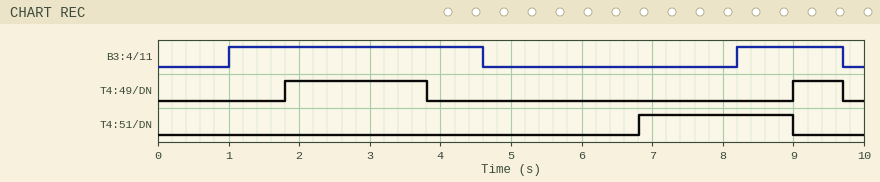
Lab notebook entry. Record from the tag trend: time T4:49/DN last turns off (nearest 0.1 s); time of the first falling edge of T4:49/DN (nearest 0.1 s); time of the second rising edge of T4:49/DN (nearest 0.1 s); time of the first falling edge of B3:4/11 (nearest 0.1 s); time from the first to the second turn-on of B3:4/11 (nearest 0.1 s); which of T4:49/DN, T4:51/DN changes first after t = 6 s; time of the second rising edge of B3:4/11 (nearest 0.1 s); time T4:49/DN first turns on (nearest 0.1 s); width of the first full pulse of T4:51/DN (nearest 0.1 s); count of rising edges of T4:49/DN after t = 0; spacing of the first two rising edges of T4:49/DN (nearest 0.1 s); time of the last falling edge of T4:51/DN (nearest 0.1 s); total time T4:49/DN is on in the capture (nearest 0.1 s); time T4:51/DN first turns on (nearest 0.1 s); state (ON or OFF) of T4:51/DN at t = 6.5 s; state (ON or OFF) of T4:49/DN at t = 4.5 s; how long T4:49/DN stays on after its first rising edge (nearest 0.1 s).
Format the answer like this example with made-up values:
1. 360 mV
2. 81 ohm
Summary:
1. 9.7 s
2. 3.8 s
3. 9.0 s
4. 4.6 s
5. 7.2 s
6. T4:51/DN
7. 8.2 s
8. 1.8 s
9. 2.2 s
10. 2
11. 7.2 s
12. 9.0 s
13. 2.7 s
14. 6.8 s
15. OFF
16. OFF
17. 2.0 s
